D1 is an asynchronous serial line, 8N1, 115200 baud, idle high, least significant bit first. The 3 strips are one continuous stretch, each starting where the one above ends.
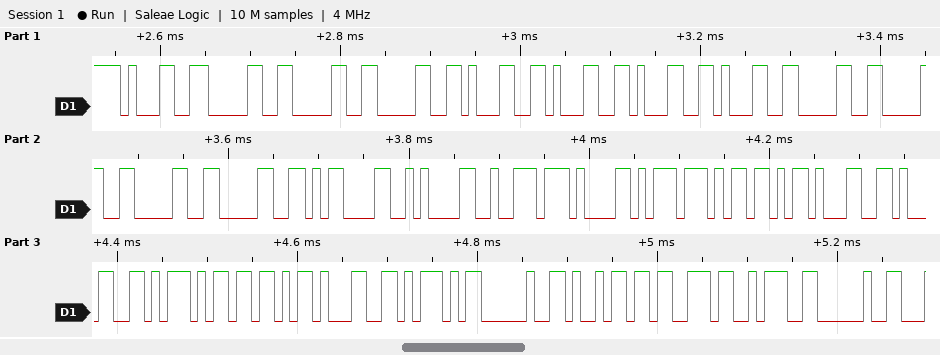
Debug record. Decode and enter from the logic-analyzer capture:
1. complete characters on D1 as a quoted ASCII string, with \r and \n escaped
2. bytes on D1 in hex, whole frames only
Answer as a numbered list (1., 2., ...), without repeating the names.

1. "100011110000\r\nraw[11][1] is: "
2. 31 30 30 30 31 31 31 31 30 30 30 30 0D 0A 72 61 77 5B 31 31 5D 5B 31 5D 20 69 73 3A 20
